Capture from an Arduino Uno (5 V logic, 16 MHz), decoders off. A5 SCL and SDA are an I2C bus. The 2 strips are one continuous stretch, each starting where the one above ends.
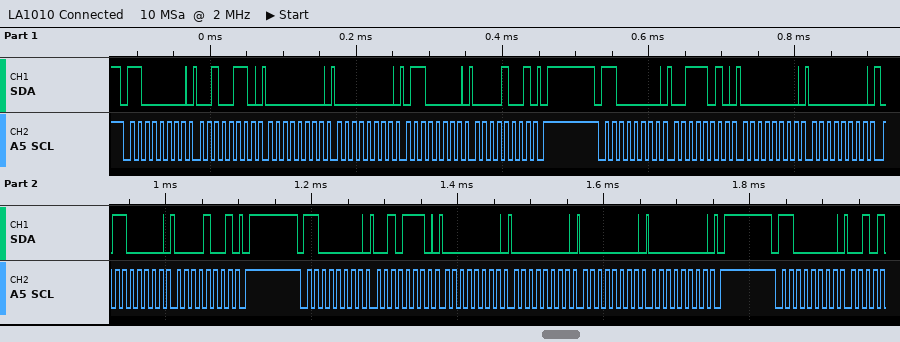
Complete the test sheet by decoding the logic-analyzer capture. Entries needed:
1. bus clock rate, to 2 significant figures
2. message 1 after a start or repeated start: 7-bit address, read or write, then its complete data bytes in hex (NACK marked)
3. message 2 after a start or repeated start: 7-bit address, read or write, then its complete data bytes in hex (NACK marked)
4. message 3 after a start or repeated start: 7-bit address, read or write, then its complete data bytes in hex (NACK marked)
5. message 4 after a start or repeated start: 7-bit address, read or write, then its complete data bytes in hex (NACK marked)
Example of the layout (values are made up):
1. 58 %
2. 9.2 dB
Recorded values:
1. 100 kHz
2. 0x60 write: 26 00 00 60 09
3. 0x60 write: 3A 00 00 60 09
4. 0x60 write: 2E 00 00 00 00
5. 0x60 write
